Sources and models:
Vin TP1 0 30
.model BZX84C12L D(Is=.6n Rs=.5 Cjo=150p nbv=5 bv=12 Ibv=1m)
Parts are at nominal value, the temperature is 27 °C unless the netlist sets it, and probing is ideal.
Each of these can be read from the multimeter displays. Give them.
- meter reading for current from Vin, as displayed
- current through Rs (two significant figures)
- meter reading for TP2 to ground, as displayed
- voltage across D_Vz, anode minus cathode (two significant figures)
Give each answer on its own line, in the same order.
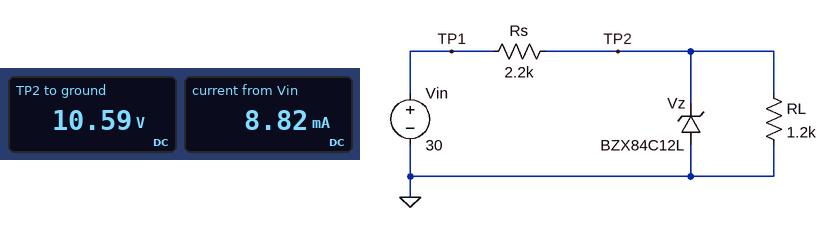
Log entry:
8.82 mA
8.8 mA
10.59 V
-11 V
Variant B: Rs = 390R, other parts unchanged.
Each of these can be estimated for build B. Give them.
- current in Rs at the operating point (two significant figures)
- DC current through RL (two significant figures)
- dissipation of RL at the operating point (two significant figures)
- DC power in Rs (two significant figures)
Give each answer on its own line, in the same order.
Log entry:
45 mA
10 mA
130 mW
790 mW
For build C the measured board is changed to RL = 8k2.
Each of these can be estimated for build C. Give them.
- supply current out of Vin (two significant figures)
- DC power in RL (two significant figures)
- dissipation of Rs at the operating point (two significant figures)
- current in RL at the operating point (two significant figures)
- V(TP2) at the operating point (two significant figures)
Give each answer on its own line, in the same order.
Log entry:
8.1 mA
18 mW
140 mW
1.5 mA
12 V
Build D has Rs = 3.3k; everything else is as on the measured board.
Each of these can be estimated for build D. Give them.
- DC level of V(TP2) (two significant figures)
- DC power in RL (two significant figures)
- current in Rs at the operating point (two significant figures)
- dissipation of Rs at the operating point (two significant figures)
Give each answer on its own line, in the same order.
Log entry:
8.0 V
53 mW
6.7 mA
150 mW
